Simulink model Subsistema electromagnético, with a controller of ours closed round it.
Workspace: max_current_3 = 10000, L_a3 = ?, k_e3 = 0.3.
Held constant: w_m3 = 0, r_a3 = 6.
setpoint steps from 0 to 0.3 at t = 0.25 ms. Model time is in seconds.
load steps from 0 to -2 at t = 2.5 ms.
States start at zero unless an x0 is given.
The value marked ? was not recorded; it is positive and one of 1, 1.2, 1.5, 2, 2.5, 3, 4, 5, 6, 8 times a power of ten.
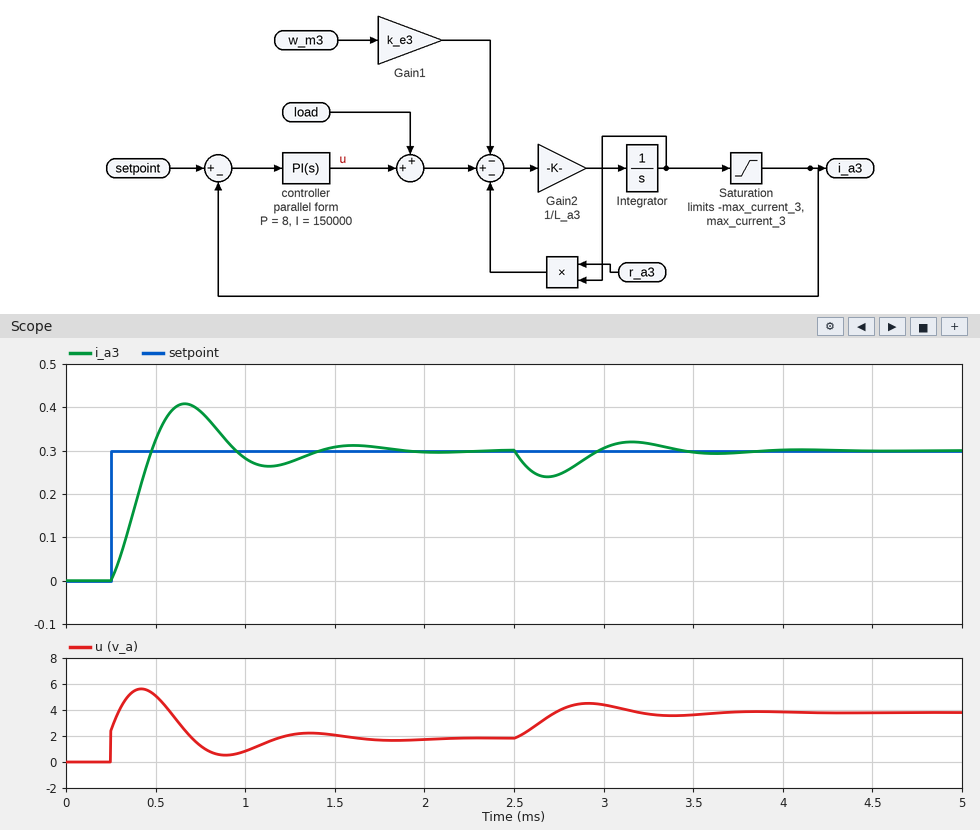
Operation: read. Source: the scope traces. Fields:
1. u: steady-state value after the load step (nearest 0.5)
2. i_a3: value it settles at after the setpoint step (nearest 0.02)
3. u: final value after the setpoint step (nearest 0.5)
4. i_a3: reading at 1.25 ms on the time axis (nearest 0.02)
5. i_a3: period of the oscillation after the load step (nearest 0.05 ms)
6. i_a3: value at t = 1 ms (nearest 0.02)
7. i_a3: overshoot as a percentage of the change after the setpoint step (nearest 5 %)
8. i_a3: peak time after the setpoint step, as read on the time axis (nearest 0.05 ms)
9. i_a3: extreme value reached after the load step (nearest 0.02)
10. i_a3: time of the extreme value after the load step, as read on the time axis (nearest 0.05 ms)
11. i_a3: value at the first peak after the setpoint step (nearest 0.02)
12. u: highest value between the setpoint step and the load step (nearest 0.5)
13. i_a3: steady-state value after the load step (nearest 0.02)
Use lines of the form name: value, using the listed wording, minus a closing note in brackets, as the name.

u: steady-state value after the load step: 4.0
i_a3: value it settles at after the setpoint step: 0.30
u: final value after the setpoint step: 2.0
i_a3: reading at 1.25 ms on the time axis: 0.28
i_a3: period of the oscillation after the load step: 0.95 ms
i_a3: value at t = 1 ms: 0.28
i_a3: overshoot as a percentage of the change after the setpoint step: 35 %
i_a3: peak time after the setpoint step, as read on the time axis: 0.65 ms
i_a3: extreme value reached after the load step: 0.24
i_a3: time of the extreme value after the load step, as read on the time axis: 2.70 ms
i_a3: value at the first peak after the setpoint step: 0.40
u: highest value between the setpoint step and the load step: 5.5
i_a3: steady-state value after the load step: 0.30
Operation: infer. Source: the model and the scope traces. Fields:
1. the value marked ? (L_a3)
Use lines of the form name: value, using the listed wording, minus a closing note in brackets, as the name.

the value marked ?: 0.003
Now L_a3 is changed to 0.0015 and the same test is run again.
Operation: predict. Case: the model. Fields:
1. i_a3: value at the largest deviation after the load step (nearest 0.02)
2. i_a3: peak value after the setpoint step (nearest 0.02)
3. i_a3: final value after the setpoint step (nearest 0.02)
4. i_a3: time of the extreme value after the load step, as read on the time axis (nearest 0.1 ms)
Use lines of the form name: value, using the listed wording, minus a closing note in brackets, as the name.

i_a3: value at the largest deviation after the load step: 0.22
i_a3: peak value after the setpoint step: 0.36
i_a3: final value after the setpoint step: 0.30
i_a3: time of the extreme value after the load step, as read on the time axis: 2.6 ms
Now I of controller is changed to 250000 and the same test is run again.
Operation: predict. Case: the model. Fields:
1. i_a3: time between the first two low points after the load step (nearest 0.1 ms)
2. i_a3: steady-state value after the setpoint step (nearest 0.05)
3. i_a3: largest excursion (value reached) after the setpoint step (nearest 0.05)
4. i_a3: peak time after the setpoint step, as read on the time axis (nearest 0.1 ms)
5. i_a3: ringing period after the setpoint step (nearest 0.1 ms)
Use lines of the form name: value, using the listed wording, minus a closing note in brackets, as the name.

i_a3: time between the first two low points after the load step: 0.7 ms
i_a3: steady-state value after the setpoint step: 0.30
i_a3: largest excursion (value reached) after the setpoint step: 0.45
i_a3: peak time after the setpoint step, as read on the time axis: 0.6 ms
i_a3: ringing period after the setpoint step: 0.7 ms
